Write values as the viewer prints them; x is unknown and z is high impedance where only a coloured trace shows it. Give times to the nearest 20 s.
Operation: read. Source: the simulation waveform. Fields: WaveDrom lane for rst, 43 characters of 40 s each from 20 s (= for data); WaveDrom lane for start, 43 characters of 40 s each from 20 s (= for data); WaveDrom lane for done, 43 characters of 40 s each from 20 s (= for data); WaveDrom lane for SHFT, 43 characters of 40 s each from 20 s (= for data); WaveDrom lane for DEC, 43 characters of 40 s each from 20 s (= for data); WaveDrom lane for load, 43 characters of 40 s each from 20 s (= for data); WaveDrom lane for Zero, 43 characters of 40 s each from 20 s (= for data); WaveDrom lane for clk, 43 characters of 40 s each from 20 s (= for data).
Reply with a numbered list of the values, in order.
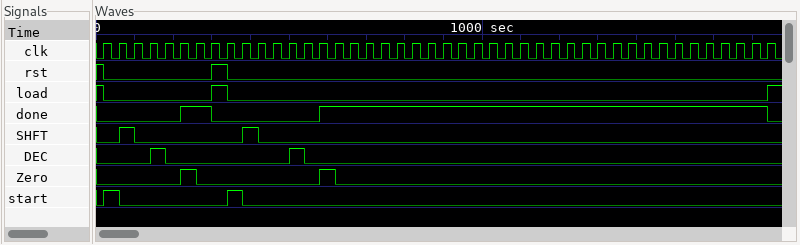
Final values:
1. {name: 'rst', wave: '0......10..................................'}
2. {name: 'start', wave: '10......10.................................'}
3. {name: 'done', wave: '0....1.0......1............................'}
4. {name: 'SHFT', wave: '010......10................................'}
5. {name: 'DEC', wave: '0..10.......10.............................'}
6. {name: 'load', wave: '0......10..................................'}
7. {name: 'Zero', wave: '0....10.......10...........................'}
8. {name: 'clk', wave: 'p..........................................'}
